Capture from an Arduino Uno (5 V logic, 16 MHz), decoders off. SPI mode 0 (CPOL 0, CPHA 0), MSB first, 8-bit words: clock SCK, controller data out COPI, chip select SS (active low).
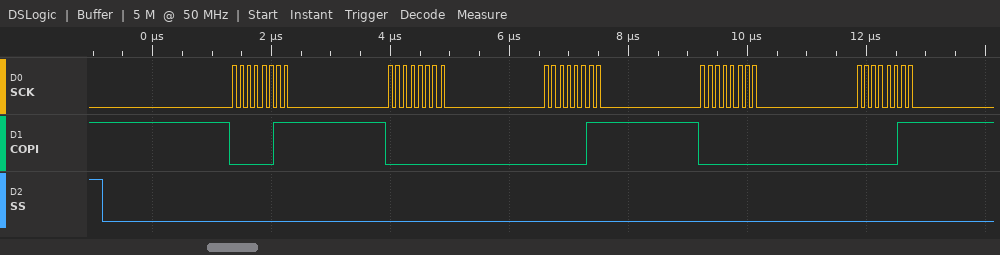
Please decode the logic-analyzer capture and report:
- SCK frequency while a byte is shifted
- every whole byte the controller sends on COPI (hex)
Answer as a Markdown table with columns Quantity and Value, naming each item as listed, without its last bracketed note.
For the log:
| Quantity | Value |
|---|---|
| SCK frequency while a byte is shifted | 8 MHz |
| every whole byte the controller sends on COPI | 03 00 03 00 03 |
